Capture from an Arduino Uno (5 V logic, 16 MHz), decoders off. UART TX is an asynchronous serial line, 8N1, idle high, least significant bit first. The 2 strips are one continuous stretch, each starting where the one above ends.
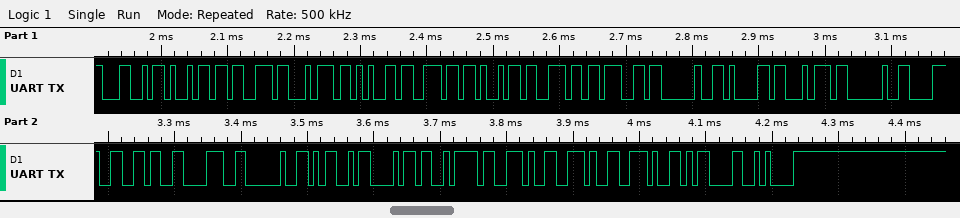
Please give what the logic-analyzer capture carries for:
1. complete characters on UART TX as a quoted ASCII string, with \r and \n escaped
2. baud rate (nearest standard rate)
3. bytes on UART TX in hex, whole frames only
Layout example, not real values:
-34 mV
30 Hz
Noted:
"Listening at 868 Mhz...\r\n"
115200 baud
4C 69 73 74 65 6E 69 6E 67 20 61 74 20 38 36 38 20 4D 68 7A 2E 2E 2E 0D 0A
